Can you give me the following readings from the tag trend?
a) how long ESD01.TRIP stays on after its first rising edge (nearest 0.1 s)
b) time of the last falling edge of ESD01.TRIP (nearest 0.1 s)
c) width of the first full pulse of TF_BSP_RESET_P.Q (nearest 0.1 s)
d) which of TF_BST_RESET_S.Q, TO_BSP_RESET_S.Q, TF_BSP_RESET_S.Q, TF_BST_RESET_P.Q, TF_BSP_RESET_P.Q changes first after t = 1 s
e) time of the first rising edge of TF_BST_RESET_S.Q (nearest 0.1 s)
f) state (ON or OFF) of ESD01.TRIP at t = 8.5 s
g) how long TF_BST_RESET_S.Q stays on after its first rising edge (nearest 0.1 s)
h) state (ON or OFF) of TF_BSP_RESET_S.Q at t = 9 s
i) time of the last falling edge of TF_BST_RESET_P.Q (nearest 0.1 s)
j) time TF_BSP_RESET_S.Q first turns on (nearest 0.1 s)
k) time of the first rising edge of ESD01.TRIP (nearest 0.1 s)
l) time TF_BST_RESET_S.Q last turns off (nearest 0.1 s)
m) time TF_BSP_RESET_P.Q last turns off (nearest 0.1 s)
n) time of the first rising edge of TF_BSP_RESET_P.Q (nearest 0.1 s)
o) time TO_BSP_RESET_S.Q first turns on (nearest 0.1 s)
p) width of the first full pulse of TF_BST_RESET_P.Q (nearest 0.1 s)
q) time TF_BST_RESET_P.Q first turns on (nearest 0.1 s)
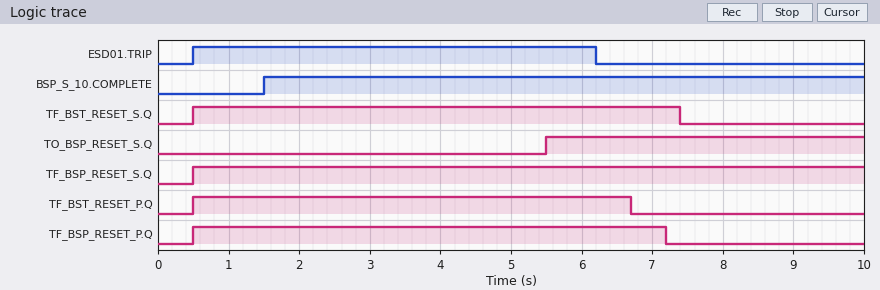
5.7 s
6.2 s
6.7 s
TO_BSP_RESET_S.Q
0.5 s
OFF
6.9 s
ON
6.7 s
0.5 s
0.5 s
7.4 s
7.2 s
0.5 s
5.5 s
6.2 s
0.5 s
